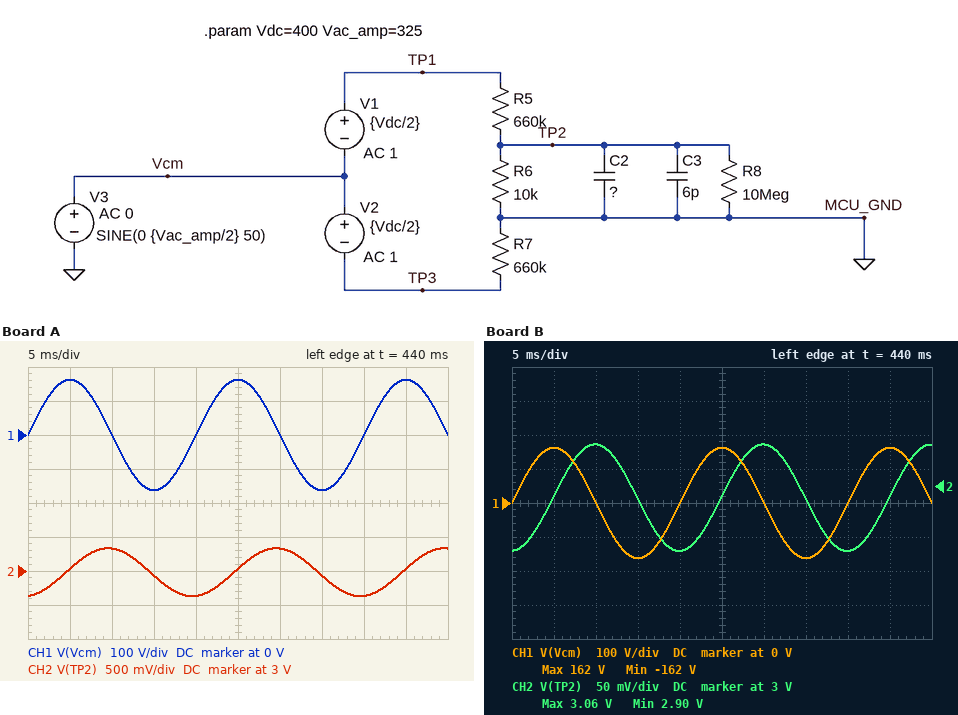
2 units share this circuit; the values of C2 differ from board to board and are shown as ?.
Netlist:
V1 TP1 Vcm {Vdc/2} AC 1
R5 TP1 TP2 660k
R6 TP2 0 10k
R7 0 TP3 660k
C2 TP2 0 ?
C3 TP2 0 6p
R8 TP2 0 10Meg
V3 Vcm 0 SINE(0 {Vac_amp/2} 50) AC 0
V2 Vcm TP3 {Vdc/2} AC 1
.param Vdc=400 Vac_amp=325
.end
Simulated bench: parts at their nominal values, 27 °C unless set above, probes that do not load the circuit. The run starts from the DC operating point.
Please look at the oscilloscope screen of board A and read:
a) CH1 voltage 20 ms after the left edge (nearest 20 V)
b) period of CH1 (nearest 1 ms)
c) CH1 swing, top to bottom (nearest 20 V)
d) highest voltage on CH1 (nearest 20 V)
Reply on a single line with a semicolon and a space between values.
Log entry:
0 V; 20 ms; 320 V; 160 V
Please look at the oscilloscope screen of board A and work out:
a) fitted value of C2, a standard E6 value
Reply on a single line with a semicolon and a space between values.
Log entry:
2.2 µF
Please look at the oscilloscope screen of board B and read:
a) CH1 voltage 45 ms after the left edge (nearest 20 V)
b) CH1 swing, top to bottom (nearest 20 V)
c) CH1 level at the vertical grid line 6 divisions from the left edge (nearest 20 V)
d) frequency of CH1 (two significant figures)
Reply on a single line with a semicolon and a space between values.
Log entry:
160 V; 320 V; 0 V; 50 Hz
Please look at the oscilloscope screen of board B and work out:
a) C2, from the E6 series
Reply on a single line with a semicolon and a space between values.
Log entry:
10 µF
